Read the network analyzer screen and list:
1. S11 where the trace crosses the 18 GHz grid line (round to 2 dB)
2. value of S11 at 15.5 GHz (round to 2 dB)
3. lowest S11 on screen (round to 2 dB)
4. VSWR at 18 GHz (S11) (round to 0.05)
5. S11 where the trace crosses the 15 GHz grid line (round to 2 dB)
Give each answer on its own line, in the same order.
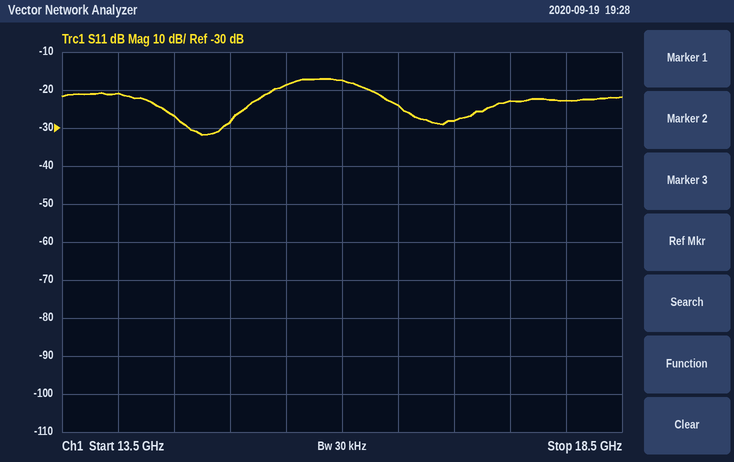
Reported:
-22 dB
-18 dB
-32 dB
1.15
-28 dB
